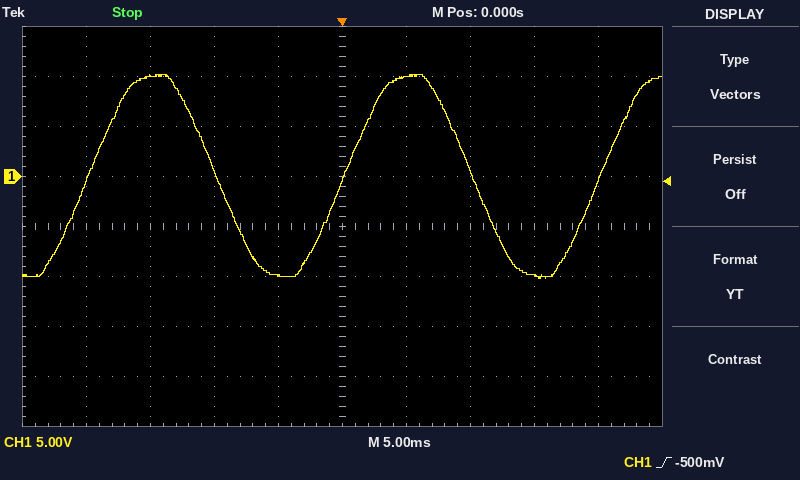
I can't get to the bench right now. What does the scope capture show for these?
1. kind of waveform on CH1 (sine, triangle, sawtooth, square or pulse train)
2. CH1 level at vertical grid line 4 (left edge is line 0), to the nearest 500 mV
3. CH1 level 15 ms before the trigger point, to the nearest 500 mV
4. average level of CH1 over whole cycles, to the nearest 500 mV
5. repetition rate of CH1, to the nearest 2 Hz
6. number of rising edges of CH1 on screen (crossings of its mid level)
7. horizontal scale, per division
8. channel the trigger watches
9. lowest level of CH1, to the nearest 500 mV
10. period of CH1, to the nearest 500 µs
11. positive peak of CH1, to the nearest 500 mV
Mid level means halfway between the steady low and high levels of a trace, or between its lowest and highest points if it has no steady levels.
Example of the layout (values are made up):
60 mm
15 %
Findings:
sine
-10.0 V
10.0 V
0.0 V
50 Hz
3
5 ms
CH1
-10.0 V
20.0 ms
10.0 V
